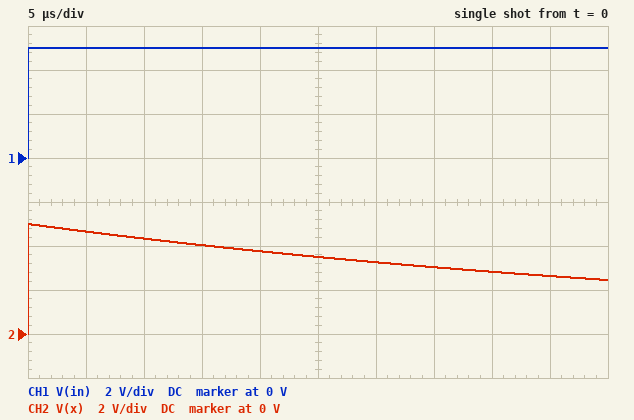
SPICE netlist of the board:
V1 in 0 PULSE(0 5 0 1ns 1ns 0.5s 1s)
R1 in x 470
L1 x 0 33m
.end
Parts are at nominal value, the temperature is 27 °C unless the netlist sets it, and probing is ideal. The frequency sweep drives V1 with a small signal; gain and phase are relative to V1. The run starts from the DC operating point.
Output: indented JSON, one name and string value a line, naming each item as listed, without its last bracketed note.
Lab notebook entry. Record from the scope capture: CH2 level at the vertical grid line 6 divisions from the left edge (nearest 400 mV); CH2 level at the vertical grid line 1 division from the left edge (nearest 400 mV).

{
  "CH2 level at the vertical grid line 6 divisions from the left edge": "3.2 V",
  "CH2 level at the vertical grid line 1 division from the left edge": "4.8 V"
}
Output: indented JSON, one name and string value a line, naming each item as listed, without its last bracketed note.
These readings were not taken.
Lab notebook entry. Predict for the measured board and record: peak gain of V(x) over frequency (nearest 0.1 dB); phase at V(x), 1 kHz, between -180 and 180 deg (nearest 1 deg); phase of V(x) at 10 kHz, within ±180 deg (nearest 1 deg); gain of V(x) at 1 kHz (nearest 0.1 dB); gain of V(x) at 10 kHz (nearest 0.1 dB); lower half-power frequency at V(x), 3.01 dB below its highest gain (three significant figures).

{
  "peak gain of V(x) over frequency": "0 dB",
  "phase at V(x), 1 kHz, between -180 and 180 deg": "66 deg",
  "phase of V(x) at 10 kHz, within ±180 deg": "13 deg",
  "gain of V(x) at 1 kHz": "-7.9 dB",
  "gain of V(x) at 10 kHz": "-0.2 dB",
  "lower half-power frequency at V(x), 3.01 dB below its highest gain": "2.27 kHz"
}
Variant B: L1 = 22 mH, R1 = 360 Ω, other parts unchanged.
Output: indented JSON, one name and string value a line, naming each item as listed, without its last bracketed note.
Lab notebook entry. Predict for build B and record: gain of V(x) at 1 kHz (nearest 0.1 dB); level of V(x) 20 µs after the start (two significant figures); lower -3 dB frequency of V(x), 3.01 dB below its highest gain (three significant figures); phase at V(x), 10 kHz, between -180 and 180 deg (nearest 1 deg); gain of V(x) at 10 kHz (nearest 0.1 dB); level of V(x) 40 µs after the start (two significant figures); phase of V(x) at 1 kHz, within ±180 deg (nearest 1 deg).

{
  "gain of V(x) at 1 kHz": "-8.9 dB",
  "level of V(x) 20 µs after the start": "3.6 V",
  "lower -3 dB frequency of V(x), 3.01 dB below its highest gain": "2.60 kHz",
  "phase at V(x), 10 kHz, between -180 and 180 deg": "15 deg",
  "gain of V(x) at 10 kHz": "-0.3 dB",
  "level of V(x) 40 µs after the start": "2.6 V",
  "phase of V(x) at 1 kHz, within ±180 deg": "69 deg"
}
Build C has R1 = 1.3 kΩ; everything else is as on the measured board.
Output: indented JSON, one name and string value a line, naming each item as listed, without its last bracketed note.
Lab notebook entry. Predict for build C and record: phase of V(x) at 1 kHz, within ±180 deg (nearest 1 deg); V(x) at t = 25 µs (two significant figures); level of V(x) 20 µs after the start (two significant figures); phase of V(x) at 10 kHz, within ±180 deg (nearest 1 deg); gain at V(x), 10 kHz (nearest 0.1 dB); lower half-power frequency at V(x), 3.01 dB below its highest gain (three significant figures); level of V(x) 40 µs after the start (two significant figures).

{
  "phase of V(x) at 1 kHz, within ±180 deg": "81 deg",
  "V(x) at t = 25 µs": "1.9 V",
  "level of V(x) 20 µs after the start": "2.3 V",
  "phase of V(x) at 10 kHz, within ±180 deg": "32 deg",
  "gain at V(x), 10 kHz": "-1.4 dB",
  "lower half-power frequency at V(x), 3.01 dB below its highest gain": "6.27 kHz",
  "level of V(x) 40 µs after the start": "1.0 V"
}
